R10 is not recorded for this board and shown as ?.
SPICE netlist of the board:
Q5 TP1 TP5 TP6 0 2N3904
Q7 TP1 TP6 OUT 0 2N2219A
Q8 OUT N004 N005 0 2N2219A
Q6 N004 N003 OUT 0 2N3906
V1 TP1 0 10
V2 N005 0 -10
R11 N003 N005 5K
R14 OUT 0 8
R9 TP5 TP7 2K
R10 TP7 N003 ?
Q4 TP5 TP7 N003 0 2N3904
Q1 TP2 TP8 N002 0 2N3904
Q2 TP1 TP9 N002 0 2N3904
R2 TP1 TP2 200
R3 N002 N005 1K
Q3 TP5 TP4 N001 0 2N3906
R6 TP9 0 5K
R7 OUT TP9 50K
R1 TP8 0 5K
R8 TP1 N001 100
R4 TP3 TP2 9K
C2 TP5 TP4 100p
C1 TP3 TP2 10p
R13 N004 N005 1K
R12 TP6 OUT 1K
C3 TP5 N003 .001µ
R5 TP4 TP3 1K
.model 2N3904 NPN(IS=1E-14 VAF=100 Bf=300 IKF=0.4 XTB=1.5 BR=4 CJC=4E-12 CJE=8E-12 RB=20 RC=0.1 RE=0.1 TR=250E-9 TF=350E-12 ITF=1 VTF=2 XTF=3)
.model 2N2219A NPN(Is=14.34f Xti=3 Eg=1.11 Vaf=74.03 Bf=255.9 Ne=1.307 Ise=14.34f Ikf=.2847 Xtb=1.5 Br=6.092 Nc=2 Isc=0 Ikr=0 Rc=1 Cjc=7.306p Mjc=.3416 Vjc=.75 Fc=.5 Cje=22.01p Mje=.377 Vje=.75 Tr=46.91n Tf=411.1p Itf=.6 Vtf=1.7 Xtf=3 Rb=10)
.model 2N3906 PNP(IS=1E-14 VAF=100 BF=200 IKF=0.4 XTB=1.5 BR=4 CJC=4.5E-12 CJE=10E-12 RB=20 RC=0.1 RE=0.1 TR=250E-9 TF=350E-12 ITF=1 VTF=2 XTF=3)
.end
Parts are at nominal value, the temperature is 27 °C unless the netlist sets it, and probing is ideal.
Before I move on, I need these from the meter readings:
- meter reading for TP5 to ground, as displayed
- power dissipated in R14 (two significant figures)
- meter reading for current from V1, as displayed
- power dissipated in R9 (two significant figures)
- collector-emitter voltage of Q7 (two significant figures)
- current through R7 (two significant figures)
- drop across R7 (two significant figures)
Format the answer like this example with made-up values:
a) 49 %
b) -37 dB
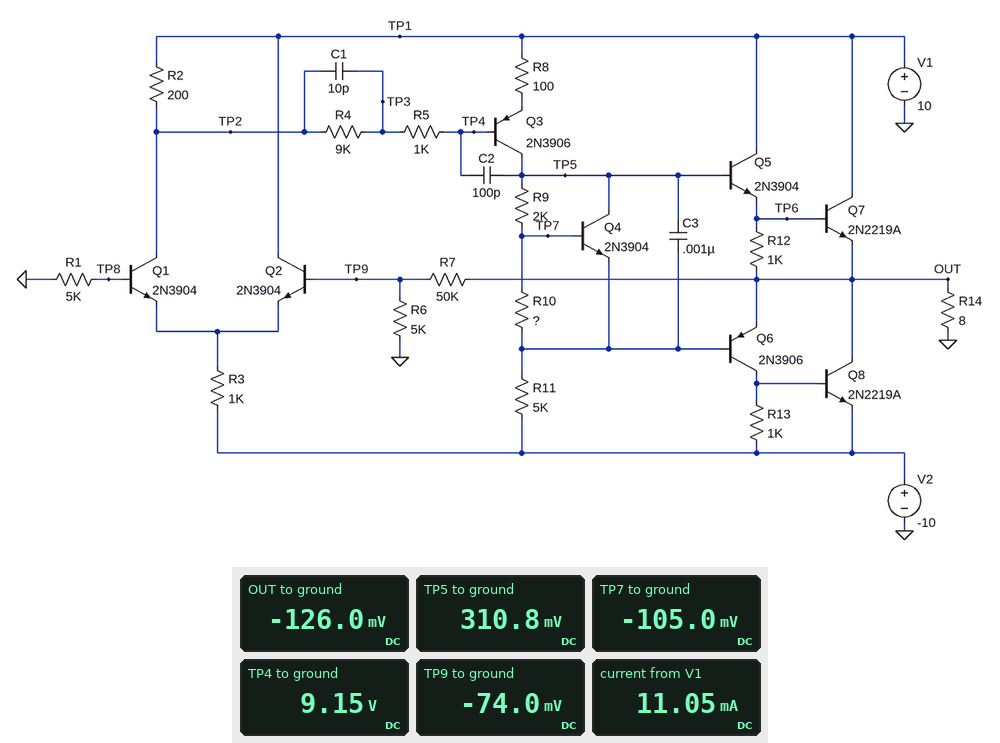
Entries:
a) 310.8 mV
b) 2.0 mW
c) 11.05 mA
d) 86 µW
e) 10 V
f) 1.0 µA
g) 52 mV
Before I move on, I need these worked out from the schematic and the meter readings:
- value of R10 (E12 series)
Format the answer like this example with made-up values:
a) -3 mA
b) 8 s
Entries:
a) 3.3 kΩ
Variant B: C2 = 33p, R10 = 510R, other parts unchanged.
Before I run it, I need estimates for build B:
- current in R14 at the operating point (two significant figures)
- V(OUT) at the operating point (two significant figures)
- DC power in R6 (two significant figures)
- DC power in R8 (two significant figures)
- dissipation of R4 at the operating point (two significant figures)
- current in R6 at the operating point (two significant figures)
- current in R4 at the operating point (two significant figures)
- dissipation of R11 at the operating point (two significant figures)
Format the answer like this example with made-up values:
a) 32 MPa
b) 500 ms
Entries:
a) 10 mA
b) -81 mV
c) 1.0 µW
d) 300 µW
e) 580 nW
f) 14 µA
g) 8.0 µA
h) 17 mW
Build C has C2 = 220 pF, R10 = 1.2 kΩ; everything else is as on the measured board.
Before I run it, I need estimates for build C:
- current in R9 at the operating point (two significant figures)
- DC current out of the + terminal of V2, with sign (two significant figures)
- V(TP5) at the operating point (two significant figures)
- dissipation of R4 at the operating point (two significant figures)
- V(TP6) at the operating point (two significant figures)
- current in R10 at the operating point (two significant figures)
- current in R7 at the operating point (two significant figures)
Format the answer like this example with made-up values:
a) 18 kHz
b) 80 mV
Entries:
a) 560 µA
b) -28 mA
c) 1.0 V
d) 660 nW
e) 360 mV
f) 550 µA
g) 1.1 µA
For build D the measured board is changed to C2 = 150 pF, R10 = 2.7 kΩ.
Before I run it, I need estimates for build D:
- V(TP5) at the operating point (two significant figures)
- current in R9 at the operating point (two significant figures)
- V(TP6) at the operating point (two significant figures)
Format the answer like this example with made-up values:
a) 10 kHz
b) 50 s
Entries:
a) 400 mV
b) 250 µA
c) -120 mV
